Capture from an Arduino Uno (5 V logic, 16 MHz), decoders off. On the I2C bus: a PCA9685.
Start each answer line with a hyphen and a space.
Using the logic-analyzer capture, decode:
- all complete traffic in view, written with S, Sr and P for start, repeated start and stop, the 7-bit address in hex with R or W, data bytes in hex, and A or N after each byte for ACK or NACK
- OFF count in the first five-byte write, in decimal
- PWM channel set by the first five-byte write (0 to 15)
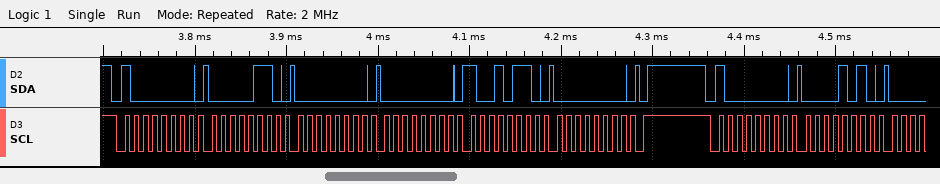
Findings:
- S 40W A 06 A 00 A 00 A 96 A 00 A P S 40W A 0A A
- 150
- 0
